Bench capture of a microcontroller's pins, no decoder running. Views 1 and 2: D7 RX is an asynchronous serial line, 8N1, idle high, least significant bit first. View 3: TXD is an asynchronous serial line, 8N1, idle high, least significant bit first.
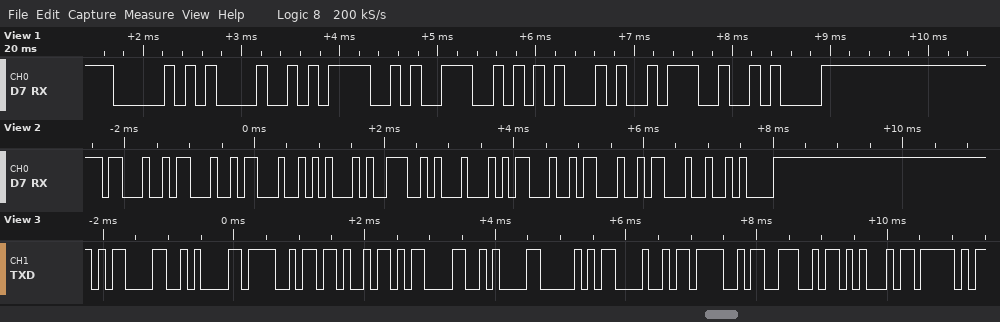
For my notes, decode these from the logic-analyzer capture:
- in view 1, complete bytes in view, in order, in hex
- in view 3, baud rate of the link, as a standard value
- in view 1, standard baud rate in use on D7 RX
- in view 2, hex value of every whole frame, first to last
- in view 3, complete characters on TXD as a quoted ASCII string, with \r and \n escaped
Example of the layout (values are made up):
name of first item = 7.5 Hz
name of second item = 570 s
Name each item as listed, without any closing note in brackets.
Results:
in view 1, complete bytes in view, in order, in hex = 50 48 4F 4E 45 3A 0A
in view 3, baud rate of the link, as a standard value = 9600 baud
in view 1, standard baud rate in use on D7 RX = 9600 baud
in view 2, hex value of every whole frame, first to last = 23 23 23 45 4E 44 23 23 23 0A
in view 3, complete characters on TXD as a quoted ASCII string, with \r and \n escaped = "\r\nOK\r\nPHONE_"
